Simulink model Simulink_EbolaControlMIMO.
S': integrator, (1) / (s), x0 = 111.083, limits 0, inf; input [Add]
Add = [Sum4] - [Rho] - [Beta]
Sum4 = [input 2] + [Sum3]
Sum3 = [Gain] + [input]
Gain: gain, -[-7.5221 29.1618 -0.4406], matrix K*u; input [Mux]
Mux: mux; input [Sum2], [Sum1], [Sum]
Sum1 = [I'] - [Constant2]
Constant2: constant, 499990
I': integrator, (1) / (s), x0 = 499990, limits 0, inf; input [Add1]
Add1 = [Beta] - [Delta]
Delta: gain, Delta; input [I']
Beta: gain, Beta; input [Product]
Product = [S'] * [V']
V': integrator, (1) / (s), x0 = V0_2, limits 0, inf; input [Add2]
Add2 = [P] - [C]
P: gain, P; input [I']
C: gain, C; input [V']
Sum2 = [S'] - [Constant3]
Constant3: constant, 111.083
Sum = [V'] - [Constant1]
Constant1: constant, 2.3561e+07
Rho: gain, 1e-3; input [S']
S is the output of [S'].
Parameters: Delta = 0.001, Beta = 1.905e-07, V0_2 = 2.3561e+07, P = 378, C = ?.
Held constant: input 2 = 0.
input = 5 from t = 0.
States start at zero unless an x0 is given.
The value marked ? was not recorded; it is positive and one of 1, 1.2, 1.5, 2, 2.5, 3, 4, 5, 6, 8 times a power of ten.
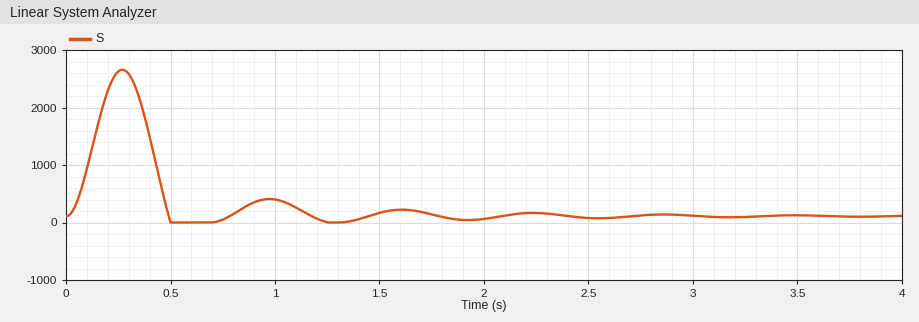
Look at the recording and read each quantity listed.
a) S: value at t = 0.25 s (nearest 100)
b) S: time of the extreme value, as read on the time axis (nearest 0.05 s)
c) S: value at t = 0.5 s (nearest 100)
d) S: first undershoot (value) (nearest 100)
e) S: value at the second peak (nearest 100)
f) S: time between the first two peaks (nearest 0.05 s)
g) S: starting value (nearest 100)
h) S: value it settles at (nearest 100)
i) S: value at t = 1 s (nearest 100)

2600
0.25 s
0
0
400
0.70 s
100
100
400
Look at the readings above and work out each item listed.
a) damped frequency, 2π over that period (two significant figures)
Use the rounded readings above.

9.0 rad/s
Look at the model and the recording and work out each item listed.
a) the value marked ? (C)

8
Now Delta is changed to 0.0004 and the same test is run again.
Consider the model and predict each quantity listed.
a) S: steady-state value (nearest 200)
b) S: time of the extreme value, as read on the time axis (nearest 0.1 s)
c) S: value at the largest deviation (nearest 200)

0
0.3 s
2600
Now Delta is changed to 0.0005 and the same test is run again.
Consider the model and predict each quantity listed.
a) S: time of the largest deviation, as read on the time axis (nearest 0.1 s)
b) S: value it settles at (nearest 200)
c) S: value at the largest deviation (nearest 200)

0.3 s
0
2600
